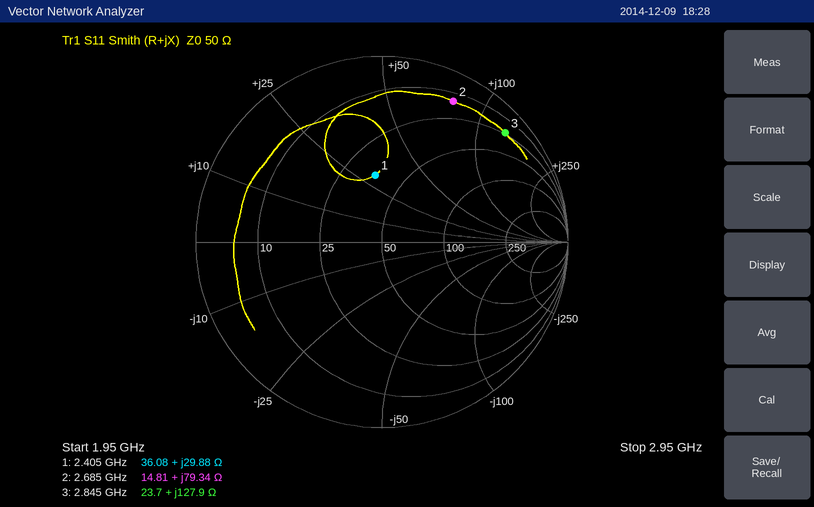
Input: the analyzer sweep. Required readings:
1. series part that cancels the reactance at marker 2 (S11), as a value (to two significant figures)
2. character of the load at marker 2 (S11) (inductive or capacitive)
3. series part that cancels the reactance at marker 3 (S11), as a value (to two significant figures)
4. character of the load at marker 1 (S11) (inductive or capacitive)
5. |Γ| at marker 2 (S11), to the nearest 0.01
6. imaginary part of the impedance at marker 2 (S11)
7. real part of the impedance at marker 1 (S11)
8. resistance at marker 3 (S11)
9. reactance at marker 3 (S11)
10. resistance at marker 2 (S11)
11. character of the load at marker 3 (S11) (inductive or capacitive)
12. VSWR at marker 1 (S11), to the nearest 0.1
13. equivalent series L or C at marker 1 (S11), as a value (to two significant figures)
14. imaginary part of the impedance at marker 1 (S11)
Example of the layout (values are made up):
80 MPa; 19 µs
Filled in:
750 fF; inductive; 440 fF; inductive; 0.85; +79.34 Ω; 36.08 Ω; 23.7 Ω; +127.9 Ω; 14.81 Ω; inductive; 2.1; 2.0 nH; +29.88 Ω
